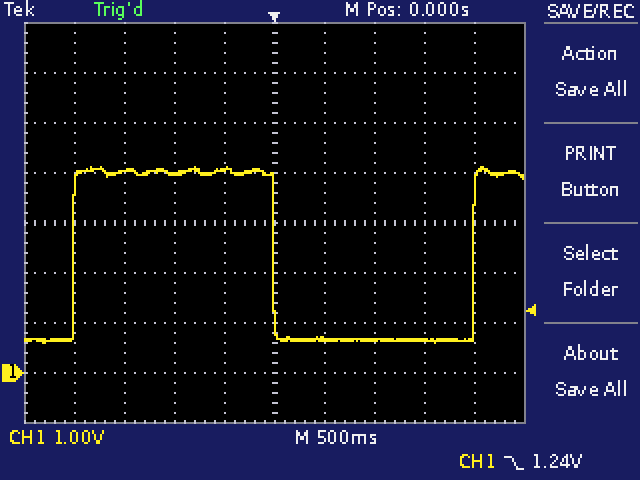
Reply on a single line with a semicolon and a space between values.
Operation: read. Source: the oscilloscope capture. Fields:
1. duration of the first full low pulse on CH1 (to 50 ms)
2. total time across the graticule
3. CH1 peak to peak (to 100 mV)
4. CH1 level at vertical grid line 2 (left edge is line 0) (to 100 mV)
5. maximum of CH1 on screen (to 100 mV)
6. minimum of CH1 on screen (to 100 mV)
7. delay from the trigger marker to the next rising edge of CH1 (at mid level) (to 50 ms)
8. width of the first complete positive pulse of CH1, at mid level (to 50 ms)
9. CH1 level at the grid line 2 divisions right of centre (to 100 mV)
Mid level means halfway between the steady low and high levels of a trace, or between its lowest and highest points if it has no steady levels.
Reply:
2.00 s; 5 s; 3.5 V; 4.0 V; 4.1 V; 600 mV; 2.00 s; 2.00 s; 700 mV
